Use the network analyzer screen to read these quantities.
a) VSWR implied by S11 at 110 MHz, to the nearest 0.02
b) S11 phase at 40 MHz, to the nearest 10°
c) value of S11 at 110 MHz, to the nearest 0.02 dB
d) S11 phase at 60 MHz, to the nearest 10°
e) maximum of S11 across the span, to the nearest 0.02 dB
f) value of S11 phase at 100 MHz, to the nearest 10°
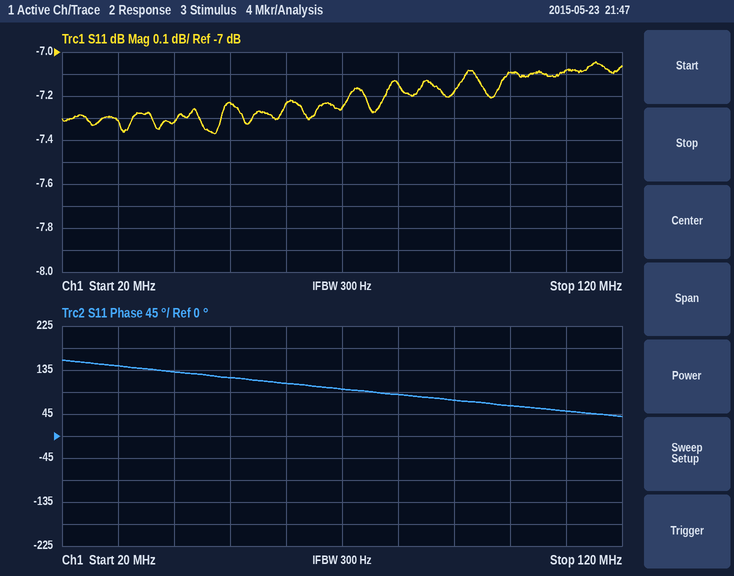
2.58
130°
-7.08 dB
110°
-7.04 dB
60°
